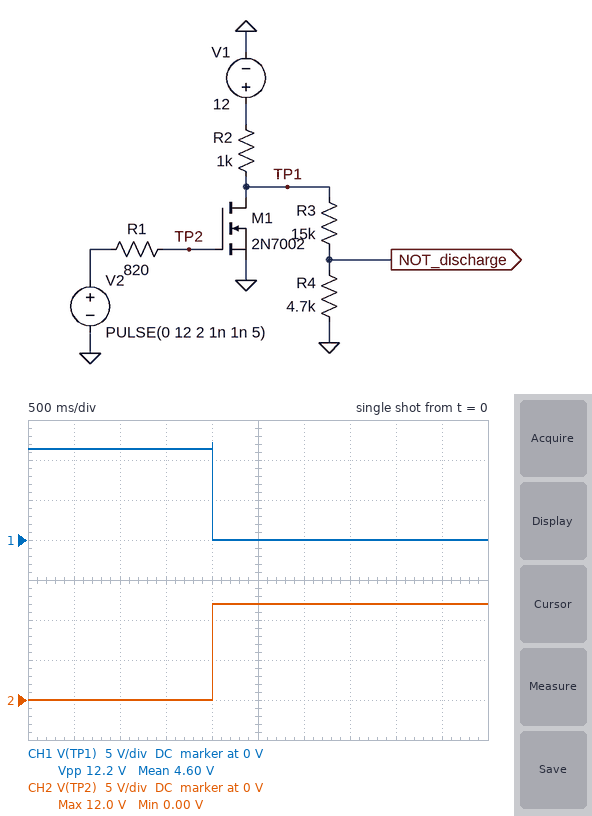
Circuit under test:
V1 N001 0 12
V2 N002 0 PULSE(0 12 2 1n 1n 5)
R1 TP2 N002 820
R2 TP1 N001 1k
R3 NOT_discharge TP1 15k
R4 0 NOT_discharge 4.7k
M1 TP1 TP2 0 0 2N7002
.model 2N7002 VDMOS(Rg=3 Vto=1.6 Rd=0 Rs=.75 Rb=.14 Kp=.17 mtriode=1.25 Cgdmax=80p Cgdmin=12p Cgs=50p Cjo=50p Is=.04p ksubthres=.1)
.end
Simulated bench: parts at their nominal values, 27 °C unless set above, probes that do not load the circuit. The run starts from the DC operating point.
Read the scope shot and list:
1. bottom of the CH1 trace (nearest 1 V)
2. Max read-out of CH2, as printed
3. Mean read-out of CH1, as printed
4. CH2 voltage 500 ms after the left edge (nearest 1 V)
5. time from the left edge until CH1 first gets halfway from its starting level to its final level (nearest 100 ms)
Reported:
0 V
12.0 V
4.60 V
0 V
2.0 s
